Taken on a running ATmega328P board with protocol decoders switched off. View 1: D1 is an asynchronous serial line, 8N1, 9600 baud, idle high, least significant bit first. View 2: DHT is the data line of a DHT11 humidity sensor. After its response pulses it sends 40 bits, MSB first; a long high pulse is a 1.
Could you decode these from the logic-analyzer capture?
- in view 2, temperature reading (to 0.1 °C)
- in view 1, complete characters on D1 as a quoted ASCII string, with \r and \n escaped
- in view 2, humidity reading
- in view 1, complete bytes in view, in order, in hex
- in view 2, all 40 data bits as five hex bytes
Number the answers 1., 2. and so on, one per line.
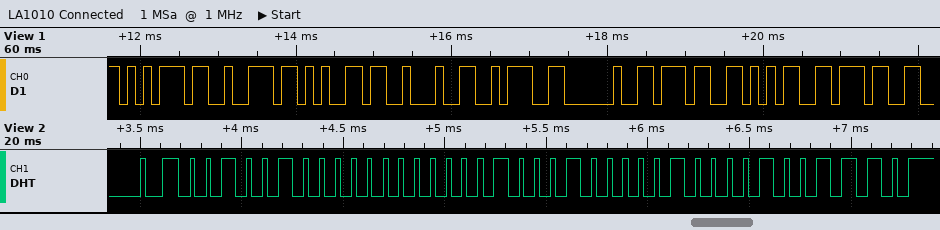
1. 34.8 °C
2. "ure\": 757"
3. 36 %
4. 75 72 65 22 3A 20 37 35 37
5. 24 00 22 08 4E
